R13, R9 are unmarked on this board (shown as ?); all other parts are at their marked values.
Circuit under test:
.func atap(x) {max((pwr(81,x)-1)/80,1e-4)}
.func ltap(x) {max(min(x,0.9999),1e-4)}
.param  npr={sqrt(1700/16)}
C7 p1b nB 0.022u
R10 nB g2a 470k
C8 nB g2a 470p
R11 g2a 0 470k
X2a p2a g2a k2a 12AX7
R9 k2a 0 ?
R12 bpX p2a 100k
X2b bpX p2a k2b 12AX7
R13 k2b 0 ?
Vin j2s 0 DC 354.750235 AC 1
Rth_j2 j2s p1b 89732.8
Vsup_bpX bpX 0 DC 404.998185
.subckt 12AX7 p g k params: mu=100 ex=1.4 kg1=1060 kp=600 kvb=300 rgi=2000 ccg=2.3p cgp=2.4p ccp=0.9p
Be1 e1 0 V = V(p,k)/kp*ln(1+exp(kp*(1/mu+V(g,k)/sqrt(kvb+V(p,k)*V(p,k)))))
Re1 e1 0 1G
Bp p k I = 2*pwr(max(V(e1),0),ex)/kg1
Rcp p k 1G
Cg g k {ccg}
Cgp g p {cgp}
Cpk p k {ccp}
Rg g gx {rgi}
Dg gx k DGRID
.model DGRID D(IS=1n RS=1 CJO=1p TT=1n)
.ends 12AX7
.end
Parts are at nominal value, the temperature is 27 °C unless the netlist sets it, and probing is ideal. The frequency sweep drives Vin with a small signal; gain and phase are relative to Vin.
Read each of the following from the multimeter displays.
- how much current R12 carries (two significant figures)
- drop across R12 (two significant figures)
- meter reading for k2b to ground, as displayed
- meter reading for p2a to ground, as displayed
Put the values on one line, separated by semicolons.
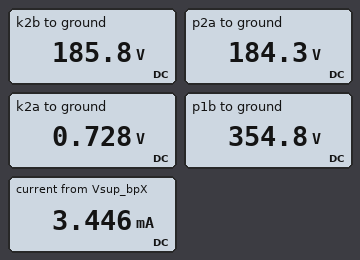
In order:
2.2 mA; 220 V; 185.8 V; 184.3 V
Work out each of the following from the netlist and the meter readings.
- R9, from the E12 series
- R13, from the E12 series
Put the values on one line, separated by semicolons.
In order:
330 Ω; 150 kΩ
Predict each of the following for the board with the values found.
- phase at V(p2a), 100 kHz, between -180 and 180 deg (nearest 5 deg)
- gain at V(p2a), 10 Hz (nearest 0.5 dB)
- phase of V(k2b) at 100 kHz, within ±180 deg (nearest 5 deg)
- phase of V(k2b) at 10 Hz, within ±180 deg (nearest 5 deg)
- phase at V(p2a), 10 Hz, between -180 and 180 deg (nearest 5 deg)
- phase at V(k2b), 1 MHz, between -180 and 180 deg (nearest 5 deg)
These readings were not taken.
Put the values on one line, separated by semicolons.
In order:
100 deg; 26.5 dB; 100 deg; -145 deg; -145 deg; 90 deg
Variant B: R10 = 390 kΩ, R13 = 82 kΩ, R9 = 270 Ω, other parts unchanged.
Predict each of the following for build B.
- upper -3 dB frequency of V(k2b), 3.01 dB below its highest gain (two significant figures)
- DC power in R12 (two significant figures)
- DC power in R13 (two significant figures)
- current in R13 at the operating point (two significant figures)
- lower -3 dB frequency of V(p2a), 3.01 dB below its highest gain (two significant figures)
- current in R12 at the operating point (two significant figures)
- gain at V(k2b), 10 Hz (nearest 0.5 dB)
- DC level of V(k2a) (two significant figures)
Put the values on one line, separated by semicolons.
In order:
19 kHz; 520 mW; 380 mW; 2.2 mA; 18 Hz; 2.3 mA; 27.5 dB; 620 mV
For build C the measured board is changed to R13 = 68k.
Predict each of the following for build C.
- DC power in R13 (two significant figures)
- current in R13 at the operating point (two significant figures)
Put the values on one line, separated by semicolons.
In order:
500 mW; 2.7 mA
